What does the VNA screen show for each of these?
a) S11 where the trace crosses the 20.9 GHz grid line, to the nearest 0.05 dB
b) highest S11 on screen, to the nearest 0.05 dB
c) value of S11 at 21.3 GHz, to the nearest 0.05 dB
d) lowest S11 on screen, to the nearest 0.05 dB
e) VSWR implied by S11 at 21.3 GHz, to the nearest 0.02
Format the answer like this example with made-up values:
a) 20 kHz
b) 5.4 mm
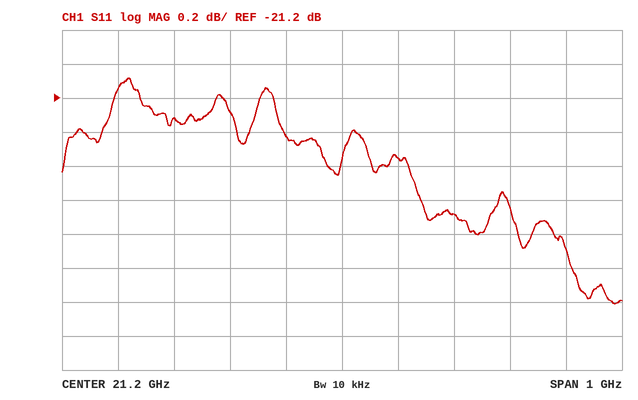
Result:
a) -21.30 dB
b) -21.10 dB
c) -21.55 dB
d) -22.40 dB
e) 1.18
